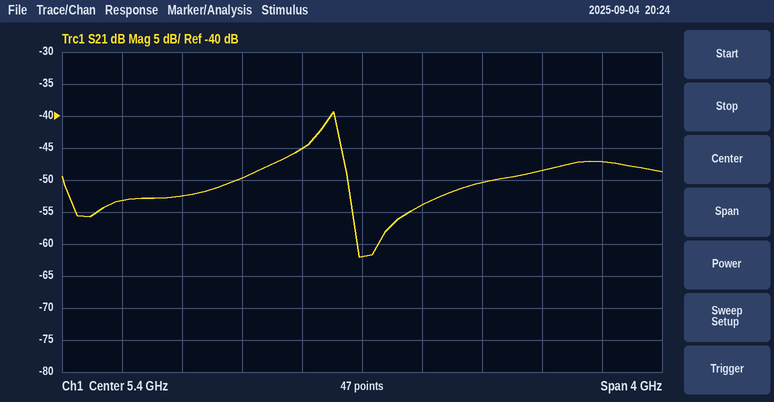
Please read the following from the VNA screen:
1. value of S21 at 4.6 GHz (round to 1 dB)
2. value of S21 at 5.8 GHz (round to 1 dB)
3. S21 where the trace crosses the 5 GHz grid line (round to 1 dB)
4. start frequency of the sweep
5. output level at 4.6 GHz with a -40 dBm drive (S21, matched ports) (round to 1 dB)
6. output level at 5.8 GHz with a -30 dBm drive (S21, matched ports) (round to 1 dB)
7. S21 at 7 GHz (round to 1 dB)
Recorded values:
-50 dB
-54 dB
-45 dB
3.4 GHz
-90 dBm
-84 dBm
-47 dB
